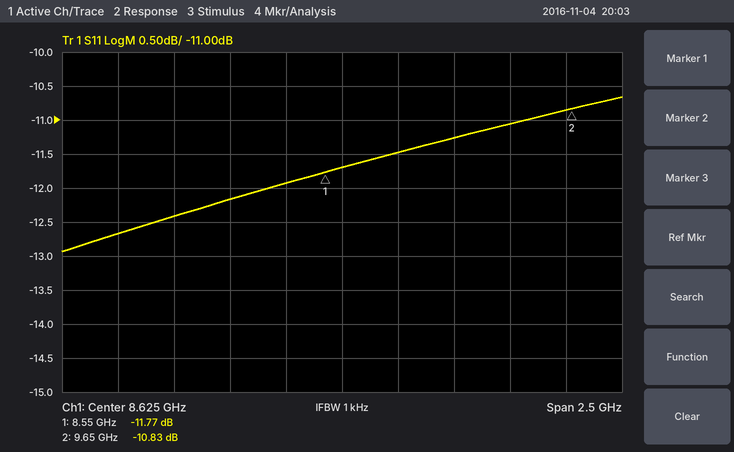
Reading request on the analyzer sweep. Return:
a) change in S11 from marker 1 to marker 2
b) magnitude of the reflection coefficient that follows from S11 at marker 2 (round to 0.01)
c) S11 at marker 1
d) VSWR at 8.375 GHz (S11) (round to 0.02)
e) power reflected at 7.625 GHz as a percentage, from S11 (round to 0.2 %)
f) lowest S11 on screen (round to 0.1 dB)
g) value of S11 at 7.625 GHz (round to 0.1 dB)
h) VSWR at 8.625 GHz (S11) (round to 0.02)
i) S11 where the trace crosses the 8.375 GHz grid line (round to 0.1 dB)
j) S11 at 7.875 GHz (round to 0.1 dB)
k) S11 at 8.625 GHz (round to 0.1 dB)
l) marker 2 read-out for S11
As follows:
0.94 dB
0.29
-11.77 dB
1.68
5.4 %
-12.9 dB
-12.7 dB
1.70
-11.9 dB
-12.4 dB
-11.7 dB
-10.83 dB
